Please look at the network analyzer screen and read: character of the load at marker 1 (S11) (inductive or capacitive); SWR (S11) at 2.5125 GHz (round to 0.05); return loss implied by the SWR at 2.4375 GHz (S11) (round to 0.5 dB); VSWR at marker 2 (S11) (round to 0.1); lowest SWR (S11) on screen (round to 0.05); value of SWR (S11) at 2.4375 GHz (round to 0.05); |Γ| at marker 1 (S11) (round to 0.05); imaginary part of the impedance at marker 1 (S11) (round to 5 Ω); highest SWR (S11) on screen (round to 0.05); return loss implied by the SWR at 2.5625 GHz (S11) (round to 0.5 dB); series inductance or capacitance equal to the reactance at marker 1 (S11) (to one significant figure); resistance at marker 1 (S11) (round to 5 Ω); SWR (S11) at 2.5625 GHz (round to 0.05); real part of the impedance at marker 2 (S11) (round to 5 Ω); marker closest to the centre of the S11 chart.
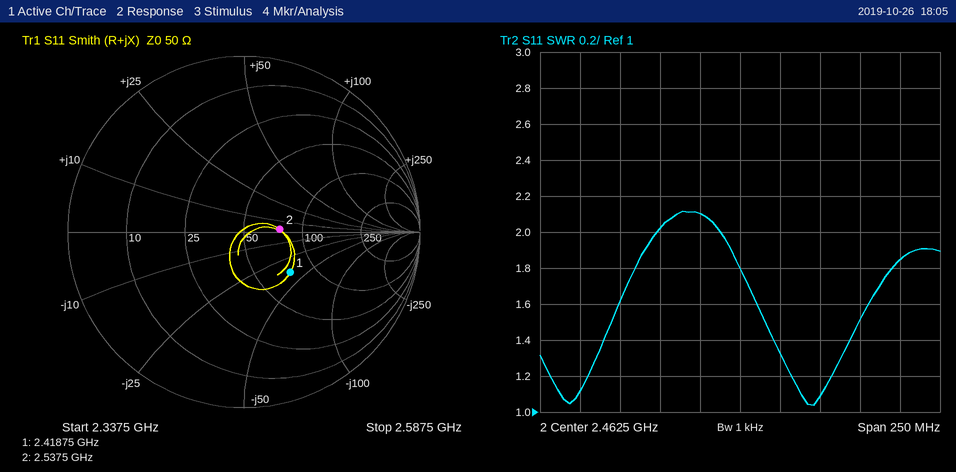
capacitive
1.10
9.0 dB
1.5
1.05
2.10
0.35
-40 Ω
2.10
10.5 dB
2 pF
75 Ω
1.85
75 Ω
marker 2
